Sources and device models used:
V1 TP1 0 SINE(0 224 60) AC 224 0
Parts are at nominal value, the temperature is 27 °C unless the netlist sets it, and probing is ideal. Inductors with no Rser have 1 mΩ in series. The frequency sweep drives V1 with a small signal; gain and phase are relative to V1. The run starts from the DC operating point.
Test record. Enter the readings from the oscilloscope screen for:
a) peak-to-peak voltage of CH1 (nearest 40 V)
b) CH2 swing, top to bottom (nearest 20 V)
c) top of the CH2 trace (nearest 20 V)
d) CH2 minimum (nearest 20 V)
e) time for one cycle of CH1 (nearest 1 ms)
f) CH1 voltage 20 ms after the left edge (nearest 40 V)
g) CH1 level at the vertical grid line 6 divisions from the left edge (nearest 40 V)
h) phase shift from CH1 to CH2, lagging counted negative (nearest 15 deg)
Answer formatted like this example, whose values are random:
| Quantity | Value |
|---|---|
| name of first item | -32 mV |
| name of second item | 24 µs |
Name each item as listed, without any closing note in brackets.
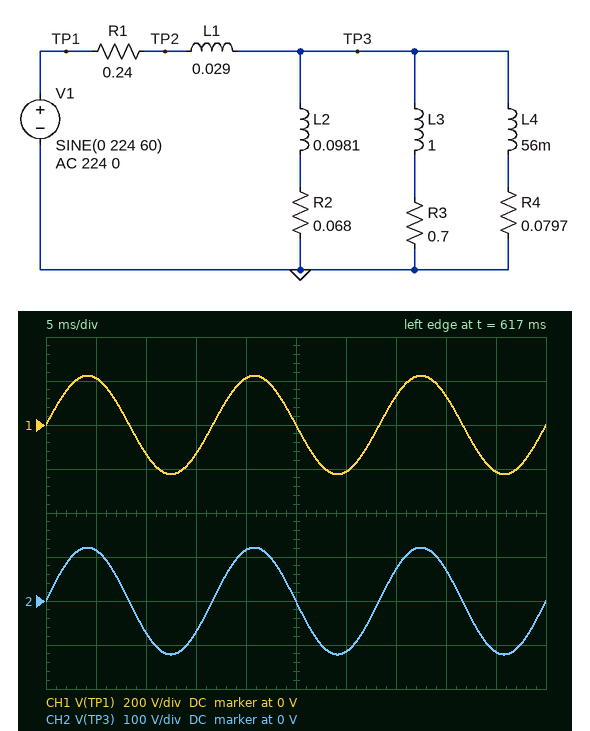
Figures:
| Quantity | Value |
|---|---|
| peak-to-peak voltage of CH1 | 440 V |
| CH2 swing, top to bottom | 240 V |
| top of the CH2 trace | 120 V |
| CH2 minimum | -120 V |
| time for one cycle of CH1 | 17 ms |
| CH1 voltage 20 ms after the left edge | 200 V |
| CH1 level at the vertical grid line 6 divisions from the left edge | -200 V |
| phase shift from CH1 to CH2, lagging counted negative | 0 deg |
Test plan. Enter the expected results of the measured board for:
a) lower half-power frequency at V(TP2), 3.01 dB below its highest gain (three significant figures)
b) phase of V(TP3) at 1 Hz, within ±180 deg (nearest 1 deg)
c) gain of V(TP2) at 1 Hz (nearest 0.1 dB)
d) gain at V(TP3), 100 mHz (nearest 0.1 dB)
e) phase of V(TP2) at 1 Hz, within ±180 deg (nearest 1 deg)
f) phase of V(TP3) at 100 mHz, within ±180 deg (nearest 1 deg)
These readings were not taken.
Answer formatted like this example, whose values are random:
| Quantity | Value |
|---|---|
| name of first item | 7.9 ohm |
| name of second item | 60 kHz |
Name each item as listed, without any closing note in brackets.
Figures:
| Quantity | Value |
|---|---|
| lower half-power frequency at V(TP2), 3.01 dB below its highest gain | 687 mHz |
| phase of V(TP3) at 1 Hz, within ±180 deg | 25 deg |
| gain of V(TP2) at 1 Hz | -1.7 dB |
| gain at V(TP3), 100 mHz | -16.2 dB |
| phase of V(TP2) at 1 Hz, within ±180 deg | 29 deg |
| phase of V(TP3) at 100 mHz, within ±180 deg | 24 deg |
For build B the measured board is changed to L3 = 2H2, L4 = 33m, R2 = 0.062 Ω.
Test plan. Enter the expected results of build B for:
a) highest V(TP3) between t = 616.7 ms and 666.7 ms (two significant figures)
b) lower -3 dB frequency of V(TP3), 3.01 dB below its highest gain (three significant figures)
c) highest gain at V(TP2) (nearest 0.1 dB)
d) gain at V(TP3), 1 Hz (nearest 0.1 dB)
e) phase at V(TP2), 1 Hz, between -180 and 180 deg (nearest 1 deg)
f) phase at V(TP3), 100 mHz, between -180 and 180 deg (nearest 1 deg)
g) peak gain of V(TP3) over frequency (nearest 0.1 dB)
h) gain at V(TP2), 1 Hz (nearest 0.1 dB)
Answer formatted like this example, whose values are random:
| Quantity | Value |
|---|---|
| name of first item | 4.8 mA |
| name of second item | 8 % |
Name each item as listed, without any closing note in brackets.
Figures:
| Quantity | Value |
|---|---|
| highest V(TP3) between t = 616.7 ms and 666.7 ms | 100 V |
| lower -3 dB frequency of V(TP3), 3.01 dB below its highest gain | 707 mHz |
| highest gain at V(TP2) | 0 dB |
| gain at V(TP3), 1 Hz | -8.7 dB |
| phase at V(TP2), 1 Hz, between -180 and 180 deg | 32 deg |
| phase at V(TP3), 100 mHz, between -180 and 180 deg | 22 deg |
| peak gain of V(TP3) over frequency | -6.8 dB |
| gain at V(TP2), 1 Hz | -2.3 dB |
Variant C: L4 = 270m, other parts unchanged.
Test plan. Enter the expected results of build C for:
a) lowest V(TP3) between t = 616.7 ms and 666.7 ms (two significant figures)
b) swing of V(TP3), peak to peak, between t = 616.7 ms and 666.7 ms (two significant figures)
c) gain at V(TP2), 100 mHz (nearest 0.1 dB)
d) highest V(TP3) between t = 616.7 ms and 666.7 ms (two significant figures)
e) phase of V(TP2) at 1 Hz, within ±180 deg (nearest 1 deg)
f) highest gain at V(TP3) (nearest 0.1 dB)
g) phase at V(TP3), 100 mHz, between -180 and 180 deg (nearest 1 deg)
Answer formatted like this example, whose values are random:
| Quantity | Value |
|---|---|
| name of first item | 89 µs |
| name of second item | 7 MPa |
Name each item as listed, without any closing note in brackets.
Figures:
| Quantity | Value |
|---|---|
| lowest V(TP3) between t = 616.7 ms and 666.7 ms | -160 V |
| swing of V(TP3), peak to peak, between t = 616.7 ms and 666.7 ms | 310 V |
| gain at V(TP2), 100 mHz | -11.7 dB |
| highest V(TP3) between t = 616.7 ms and 666.7 ms | 160 V |
| phase of V(TP2) at 1 Hz, within ±180 deg | 21 deg |
| highest gain at V(TP3) | -3.1 dB |
| phase at V(TP3), 100 mHz, between -180 and 180 deg | 36 deg |
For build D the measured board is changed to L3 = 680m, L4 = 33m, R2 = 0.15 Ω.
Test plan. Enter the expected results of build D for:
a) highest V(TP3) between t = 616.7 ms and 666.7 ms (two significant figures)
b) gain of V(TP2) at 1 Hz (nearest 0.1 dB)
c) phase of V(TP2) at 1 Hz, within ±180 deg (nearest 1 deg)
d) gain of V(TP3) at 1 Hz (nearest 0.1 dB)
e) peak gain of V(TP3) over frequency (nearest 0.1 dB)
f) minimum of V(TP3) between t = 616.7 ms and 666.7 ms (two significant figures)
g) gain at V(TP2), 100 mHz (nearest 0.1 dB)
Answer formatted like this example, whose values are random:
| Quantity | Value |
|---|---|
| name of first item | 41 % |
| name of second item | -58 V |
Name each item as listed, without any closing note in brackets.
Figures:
| Quantity | Value |
|---|---|
| highest V(TP3) between t = 616.7 ms and 666.7 ms | 100 V |
| gain of V(TP2) at 1 Hz | -2.4 dB |
| phase of V(TP2) at 1 Hz, within ±180 deg | 32 deg |
| gain of V(TP3) at 1 Hz | -8.9 dB |
| peak gain of V(TP3) over frequency | -6.9 dB |
| minimum of V(TP3) between t = 616.7 ms and 666.7 ms | -100 V |
| gain at V(TP2), 100 mHz | -13.6 dB |
